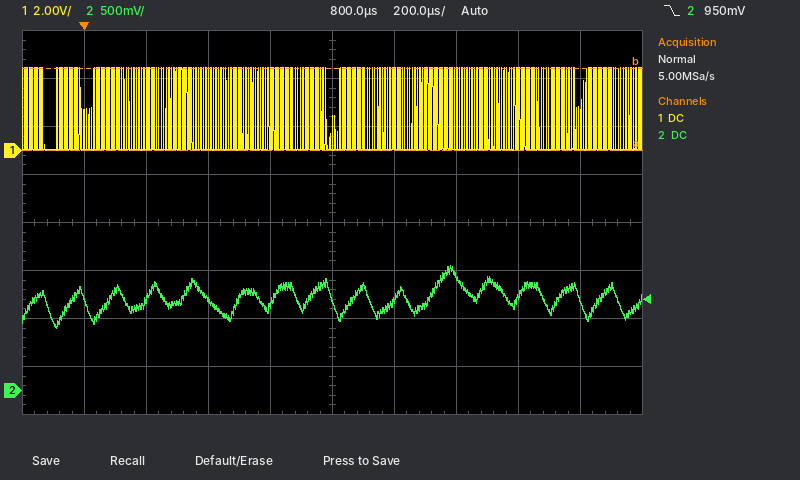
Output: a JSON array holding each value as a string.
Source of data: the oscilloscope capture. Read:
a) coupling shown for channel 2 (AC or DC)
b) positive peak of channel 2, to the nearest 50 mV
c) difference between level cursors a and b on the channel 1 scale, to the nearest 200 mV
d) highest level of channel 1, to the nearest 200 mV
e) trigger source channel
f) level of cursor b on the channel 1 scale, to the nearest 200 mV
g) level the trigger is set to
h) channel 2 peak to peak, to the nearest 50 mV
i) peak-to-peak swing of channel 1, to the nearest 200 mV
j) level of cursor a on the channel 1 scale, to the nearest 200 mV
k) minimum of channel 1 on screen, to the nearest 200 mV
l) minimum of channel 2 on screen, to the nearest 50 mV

["DC", "1.30 V", "3.4 V", "3.4 V", "channel 2", "3.4 V", "950 mV", "650 mV", "3.4 V", "0.0 V", "0.0 V", "650 mV"]
